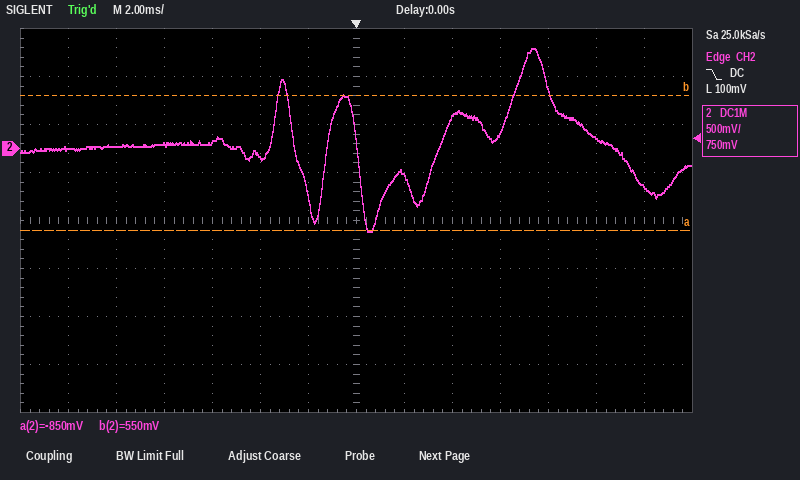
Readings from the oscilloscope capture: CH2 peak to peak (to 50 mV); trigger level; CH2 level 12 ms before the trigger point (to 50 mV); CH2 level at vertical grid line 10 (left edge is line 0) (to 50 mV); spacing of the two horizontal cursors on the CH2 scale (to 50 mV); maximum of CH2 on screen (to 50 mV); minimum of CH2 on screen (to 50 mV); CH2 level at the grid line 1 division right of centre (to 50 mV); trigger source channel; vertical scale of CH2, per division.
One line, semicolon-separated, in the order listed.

1.90 V; 100 mV; 0 mV; 150 mV; 1.40 V; 1.05 V; -850 mV; -300 mV; CH2; 500 mV
